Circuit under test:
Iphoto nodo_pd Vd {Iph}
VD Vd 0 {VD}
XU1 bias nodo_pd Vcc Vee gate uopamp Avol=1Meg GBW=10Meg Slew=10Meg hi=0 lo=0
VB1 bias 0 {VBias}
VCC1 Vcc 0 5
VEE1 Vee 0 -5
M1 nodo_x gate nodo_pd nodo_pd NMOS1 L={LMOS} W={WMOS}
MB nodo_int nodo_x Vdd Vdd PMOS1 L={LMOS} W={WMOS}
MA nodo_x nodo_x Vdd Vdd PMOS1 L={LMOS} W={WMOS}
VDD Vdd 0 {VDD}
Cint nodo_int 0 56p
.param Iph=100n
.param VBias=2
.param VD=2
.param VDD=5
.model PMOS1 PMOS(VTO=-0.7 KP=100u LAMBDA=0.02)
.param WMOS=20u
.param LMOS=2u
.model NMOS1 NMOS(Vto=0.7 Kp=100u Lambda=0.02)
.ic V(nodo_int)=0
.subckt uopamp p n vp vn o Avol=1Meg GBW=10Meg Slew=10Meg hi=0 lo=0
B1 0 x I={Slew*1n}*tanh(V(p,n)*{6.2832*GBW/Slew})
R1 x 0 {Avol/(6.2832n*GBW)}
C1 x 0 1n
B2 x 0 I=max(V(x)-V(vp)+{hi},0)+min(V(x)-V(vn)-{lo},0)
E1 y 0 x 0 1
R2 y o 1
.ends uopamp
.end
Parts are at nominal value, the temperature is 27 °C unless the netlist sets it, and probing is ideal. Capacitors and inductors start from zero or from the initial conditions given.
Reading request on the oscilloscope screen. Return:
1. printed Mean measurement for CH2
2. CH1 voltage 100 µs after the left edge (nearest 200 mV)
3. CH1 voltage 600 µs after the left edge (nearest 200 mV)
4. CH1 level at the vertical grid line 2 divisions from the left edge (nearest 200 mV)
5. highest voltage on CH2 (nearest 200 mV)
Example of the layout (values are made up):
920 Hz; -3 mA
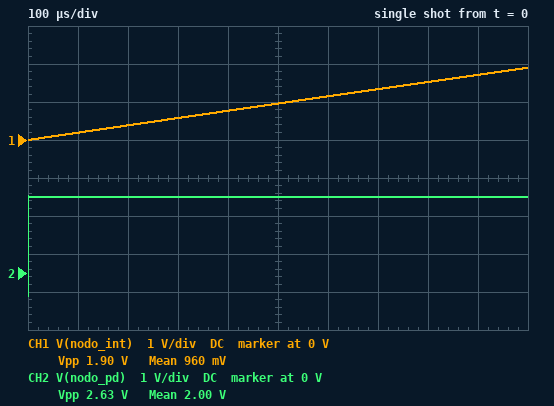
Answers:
2.00 V; 200 mV; 1.2 V; 400 mV; 2.0 V
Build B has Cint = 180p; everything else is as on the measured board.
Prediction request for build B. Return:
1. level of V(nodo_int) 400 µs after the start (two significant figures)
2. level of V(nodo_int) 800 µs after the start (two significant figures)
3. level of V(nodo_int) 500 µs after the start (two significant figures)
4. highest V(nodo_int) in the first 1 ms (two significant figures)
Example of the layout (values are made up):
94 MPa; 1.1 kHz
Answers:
240 mV; 480 mV; 300 mV; 600 mV
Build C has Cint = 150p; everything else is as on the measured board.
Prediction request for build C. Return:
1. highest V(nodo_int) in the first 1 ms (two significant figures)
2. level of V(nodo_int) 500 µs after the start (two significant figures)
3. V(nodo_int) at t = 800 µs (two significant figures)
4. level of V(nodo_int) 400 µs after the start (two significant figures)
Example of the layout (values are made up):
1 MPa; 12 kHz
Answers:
720 mV; 360 mV; 580 mV; 290 mV
